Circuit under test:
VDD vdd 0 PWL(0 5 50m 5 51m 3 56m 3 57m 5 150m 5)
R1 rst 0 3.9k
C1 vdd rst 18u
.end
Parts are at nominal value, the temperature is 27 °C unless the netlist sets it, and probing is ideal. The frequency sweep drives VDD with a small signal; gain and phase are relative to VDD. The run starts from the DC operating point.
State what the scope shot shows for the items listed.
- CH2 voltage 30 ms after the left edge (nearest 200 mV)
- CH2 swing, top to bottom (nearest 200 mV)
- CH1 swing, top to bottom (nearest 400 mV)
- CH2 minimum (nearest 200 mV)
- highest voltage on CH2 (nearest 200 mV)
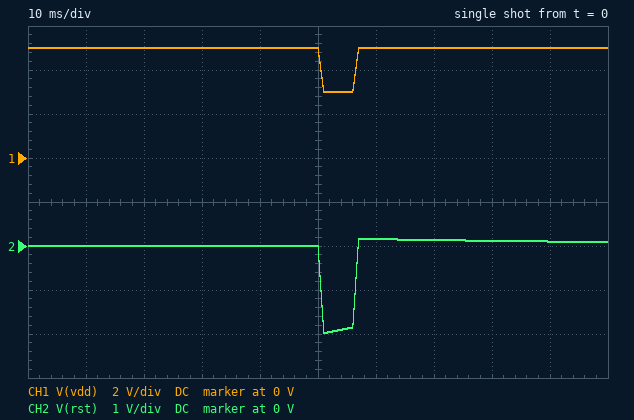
0 V
2.2 V
2.0 V
-2.0 V
200 mV
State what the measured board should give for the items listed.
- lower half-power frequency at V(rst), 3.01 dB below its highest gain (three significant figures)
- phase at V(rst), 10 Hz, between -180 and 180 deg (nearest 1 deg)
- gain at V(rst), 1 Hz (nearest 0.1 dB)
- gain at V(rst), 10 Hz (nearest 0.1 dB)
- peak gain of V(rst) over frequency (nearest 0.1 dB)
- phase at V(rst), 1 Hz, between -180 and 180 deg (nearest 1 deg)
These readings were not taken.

2.27 Hz
13 deg
-7.9 dB
-0.2 dB
0 dB
66 deg
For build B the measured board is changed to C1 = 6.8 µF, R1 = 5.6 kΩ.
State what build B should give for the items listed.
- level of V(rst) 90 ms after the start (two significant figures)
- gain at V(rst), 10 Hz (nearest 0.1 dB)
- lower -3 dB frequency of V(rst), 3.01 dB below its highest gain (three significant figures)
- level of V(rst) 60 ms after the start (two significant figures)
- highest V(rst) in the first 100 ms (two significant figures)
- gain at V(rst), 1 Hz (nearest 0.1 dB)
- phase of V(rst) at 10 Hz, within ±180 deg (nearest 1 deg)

120 mV
-0.7 dB
4.18 Hz
270 mV
290 mV
-12.7 dB
23 deg
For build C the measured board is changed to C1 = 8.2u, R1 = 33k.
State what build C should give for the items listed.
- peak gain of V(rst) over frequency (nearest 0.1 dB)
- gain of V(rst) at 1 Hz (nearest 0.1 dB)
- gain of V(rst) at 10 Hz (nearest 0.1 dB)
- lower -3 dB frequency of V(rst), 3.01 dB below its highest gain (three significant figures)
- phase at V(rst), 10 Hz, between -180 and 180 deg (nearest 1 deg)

0 dB
-1.3 dB
0 dB
588 mHz
3 deg
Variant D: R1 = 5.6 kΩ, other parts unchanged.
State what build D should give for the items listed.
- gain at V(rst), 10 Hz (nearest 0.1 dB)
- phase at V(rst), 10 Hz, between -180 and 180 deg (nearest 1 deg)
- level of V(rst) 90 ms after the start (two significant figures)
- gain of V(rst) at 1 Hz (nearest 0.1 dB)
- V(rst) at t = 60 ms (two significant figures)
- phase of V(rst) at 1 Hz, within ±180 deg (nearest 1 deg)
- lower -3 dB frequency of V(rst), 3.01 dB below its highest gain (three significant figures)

-0.1 dB
9 deg
83 mV
-5.4 dB
110 mV
58 deg
1.58 Hz
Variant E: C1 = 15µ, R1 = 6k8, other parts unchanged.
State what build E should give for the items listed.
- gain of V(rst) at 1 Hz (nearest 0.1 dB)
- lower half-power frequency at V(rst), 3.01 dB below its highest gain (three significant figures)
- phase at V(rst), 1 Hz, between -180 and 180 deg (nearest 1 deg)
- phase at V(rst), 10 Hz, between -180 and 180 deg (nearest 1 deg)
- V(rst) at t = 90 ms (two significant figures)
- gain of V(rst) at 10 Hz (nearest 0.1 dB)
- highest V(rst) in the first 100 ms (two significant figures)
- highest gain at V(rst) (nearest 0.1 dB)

-5.4 dB
1.56 Hz
57 deg
9 deg
82 mV
-0.1 dB
110 mV
0 dB
